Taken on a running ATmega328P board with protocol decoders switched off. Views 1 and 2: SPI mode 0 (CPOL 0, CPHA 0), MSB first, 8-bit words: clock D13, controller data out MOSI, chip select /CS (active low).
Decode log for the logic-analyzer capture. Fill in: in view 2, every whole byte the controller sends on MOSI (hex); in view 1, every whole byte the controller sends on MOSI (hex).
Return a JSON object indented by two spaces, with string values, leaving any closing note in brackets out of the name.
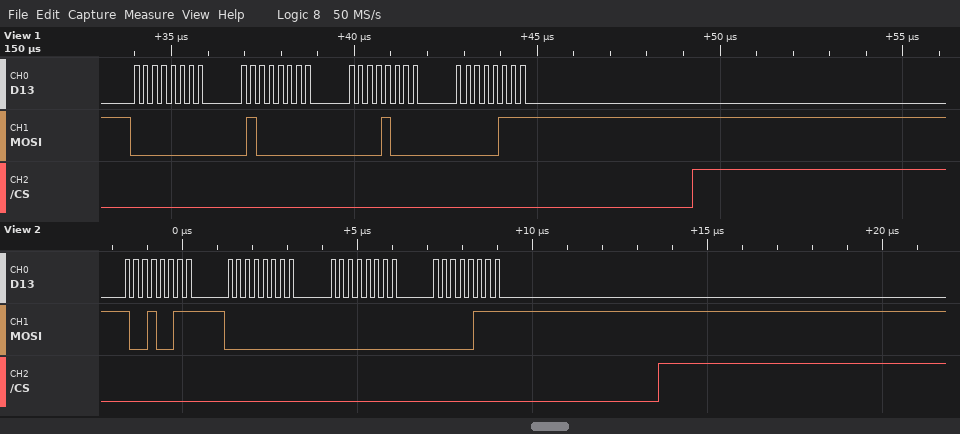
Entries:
{
  "in view 2, every whole byte the controller sends on MOSI": "93 00 00 07",
  "in view 1, every whole byte the controller sends on MOSI": "0x00 0x40 0x08 0x07"
}
